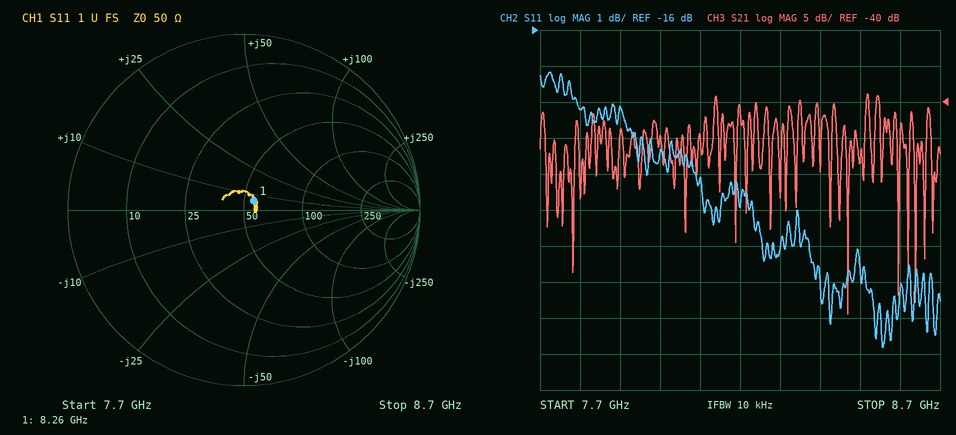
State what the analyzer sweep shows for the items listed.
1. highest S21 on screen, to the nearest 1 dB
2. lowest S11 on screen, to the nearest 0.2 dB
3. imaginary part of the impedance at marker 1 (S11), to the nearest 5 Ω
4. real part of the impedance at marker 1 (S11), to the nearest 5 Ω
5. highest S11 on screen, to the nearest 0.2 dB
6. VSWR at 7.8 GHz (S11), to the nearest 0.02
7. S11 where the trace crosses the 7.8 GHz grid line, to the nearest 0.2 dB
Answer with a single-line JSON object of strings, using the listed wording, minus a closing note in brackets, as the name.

{"highest S21 on screen, to the nearest 1 dB": "-39 dB", "lowest S11 on screen, to the nearest 0.2 dB": "-24.8 dB", "imaginary part of the impedance at marker 1 (S11), to the nearest 5 Ω": "+5 Ω", "real part of the impedance at marker 1 (S11), to the nearest 5 Ω": "55 Ω", "highest S11 on screen, to the nearest 0.2 dB": "-17.2 dB", "VSWR at 7.8 GHz (S11), to the nearest 0.02": "1.28", "S11 where the trace crosses the 7.8 GHz grid line, to the nearest 0.2 dB": "-18.2 dB"}
